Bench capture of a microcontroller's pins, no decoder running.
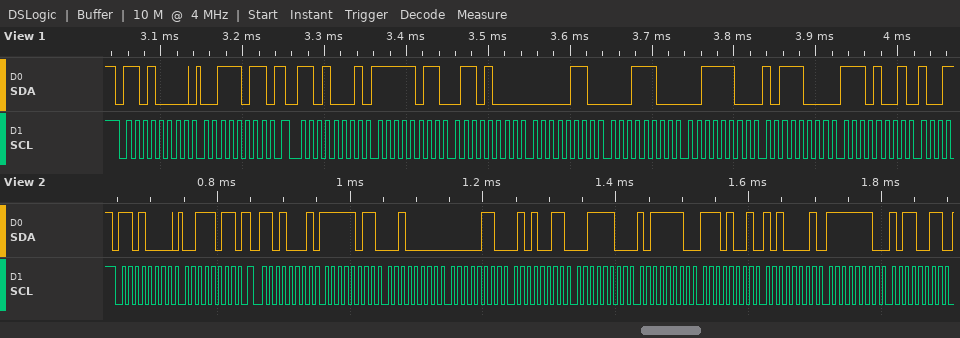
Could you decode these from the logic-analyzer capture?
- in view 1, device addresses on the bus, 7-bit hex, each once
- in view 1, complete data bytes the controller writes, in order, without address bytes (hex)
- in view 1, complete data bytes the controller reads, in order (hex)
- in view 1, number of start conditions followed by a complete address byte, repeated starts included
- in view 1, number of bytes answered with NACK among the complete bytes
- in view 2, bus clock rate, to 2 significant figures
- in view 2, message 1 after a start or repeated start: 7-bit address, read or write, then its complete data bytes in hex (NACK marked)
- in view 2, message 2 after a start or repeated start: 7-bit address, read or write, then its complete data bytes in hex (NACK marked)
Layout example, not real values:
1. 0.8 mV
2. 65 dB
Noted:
1. 0x68
2. 3B
3. FB 68 06 1C 3C B8 E9
4. 2
5. 0
6. 100 kHz
7. 0x68 write: 3B
8. 0x68 read: FB 20 06 53 3C BE E9 A1 FE B3
